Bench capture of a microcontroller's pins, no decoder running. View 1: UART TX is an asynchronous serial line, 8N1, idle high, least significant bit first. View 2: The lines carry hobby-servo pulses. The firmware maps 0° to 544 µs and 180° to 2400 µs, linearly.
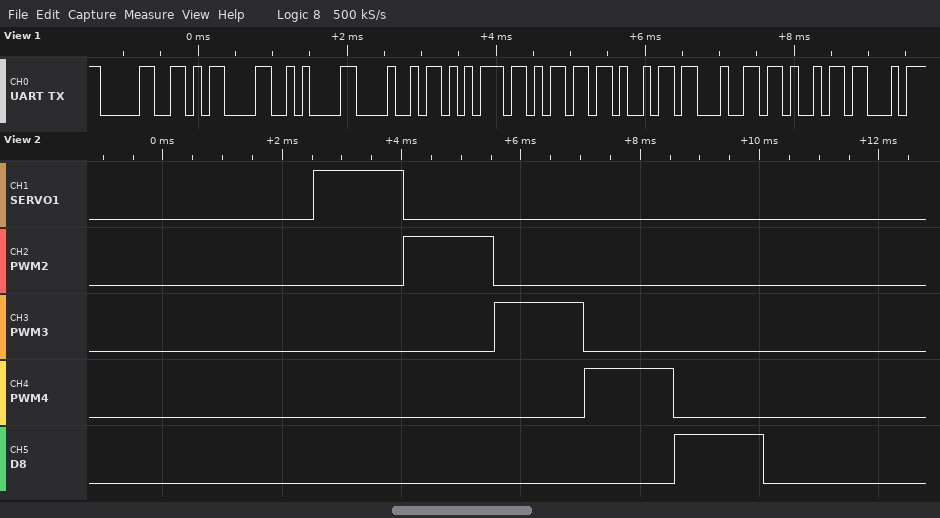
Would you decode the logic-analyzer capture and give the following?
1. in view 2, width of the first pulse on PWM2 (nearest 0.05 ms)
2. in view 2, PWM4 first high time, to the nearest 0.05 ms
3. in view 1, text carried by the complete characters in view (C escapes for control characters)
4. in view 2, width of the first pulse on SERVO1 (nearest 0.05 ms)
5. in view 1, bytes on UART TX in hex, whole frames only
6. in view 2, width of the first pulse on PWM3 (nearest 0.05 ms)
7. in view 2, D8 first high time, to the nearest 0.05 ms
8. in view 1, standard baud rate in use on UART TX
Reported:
1.50 ms
1.50 ms
"0\r\nHumidi"
1.50 ms
30 0D 0A 48 75 6D 69 64 69
1.50 ms
1.50 ms
9600 baud
